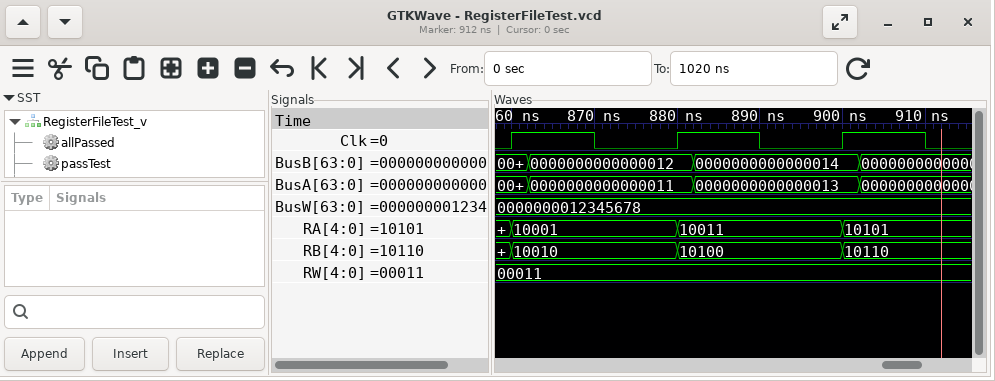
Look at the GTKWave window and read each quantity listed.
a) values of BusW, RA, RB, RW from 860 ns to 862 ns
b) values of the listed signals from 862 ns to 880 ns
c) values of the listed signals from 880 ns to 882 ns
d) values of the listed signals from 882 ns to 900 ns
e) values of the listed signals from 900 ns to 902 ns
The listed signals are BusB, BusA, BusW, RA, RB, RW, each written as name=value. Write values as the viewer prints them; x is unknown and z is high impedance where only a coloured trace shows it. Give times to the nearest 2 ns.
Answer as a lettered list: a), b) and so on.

a) BusW=0000000012345678, RA=10001, RB=10010, RW=00011
b) BusB=0000000000000012, BusA=0000000000000011, BusW=0000000012345678, RA=10001, RB=10010, RW=00011
c) BusB=0000000000000012, BusA=0000000000000011, BusW=0000000012345678, RA=10011, RB=10100, RW=00011
d) BusB=0000000000000014, BusA=0000000000000013, BusW=0000000012345678, RA=10011, RB=10100, RW=00011
e) BusB=0000000000000014, BusA=0000000000000013, BusW=0000000012345678, RA=10101, RB=10110, RW=00011
